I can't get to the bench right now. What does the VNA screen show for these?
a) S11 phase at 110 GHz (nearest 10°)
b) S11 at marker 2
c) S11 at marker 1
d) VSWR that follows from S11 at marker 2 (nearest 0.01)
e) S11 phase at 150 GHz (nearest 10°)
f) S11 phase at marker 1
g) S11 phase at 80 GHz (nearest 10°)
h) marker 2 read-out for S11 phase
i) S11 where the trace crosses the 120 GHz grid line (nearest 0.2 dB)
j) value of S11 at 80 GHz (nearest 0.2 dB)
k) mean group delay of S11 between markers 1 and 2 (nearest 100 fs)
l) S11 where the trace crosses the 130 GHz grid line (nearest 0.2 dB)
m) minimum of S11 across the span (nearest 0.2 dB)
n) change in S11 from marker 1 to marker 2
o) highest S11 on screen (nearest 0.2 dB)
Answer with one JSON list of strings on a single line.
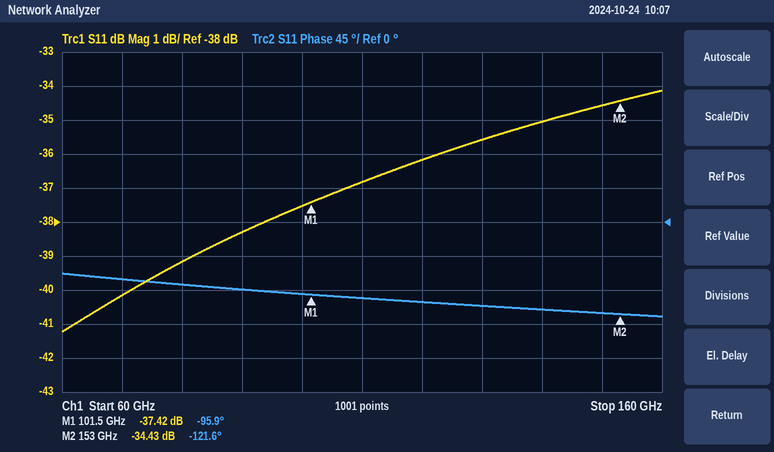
["-100°", "-34.43 dB", "-37.42 dB", "1.04", "-120°", "-95.9°", "-80°", "-121.6°", "-36.2 dB", "-39.2 dB", "1.4 ps", "-35.6 dB", "-41.2 dB", "2.99 dB", "-34.2 dB"]
